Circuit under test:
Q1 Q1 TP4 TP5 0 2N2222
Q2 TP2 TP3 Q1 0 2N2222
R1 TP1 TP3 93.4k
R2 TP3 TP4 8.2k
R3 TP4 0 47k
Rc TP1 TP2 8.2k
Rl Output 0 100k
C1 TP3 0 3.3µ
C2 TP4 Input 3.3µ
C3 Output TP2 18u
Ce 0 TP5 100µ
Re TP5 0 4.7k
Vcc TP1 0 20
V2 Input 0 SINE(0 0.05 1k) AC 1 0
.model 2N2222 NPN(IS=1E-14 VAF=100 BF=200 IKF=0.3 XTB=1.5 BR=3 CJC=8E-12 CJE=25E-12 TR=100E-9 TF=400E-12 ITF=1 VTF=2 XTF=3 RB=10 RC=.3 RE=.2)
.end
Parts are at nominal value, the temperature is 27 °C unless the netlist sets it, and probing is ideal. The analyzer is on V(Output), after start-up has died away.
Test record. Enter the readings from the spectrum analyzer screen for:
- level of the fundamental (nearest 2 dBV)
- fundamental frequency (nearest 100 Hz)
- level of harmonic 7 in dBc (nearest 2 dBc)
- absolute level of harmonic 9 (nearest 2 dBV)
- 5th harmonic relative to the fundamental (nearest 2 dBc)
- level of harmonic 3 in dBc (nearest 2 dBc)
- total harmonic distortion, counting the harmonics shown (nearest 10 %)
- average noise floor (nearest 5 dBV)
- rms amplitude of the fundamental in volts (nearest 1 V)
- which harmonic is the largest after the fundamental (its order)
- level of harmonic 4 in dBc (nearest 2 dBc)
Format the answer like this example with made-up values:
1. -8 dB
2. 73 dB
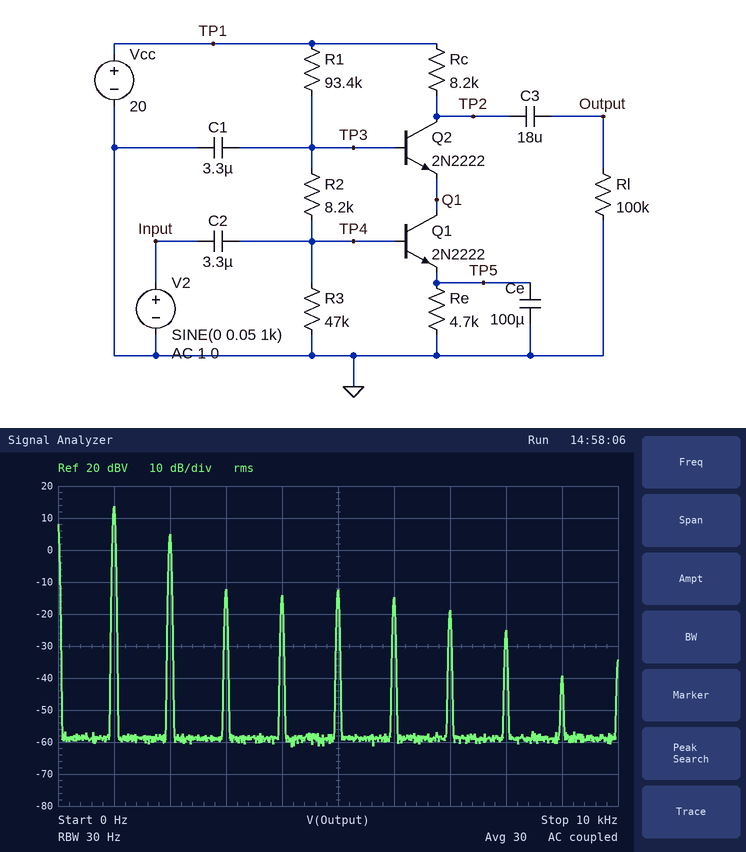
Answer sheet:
1. 14 dBV
2. 1.0 kHz
3. -32 dBc
4. -40 dBV
5. -26 dBc
6. -26 dBc
7. 40 %
8. -60 dBV
9. 5 V
10. 2
11. -28 dBc
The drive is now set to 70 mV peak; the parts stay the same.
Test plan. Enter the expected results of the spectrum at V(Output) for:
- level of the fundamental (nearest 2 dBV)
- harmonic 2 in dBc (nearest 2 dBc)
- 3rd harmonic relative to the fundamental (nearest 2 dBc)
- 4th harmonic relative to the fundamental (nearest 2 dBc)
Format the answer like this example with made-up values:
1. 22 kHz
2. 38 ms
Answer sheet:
1. 14 dBV
2. -6 dBc
3. -18 dBc
4. -34 dBc
